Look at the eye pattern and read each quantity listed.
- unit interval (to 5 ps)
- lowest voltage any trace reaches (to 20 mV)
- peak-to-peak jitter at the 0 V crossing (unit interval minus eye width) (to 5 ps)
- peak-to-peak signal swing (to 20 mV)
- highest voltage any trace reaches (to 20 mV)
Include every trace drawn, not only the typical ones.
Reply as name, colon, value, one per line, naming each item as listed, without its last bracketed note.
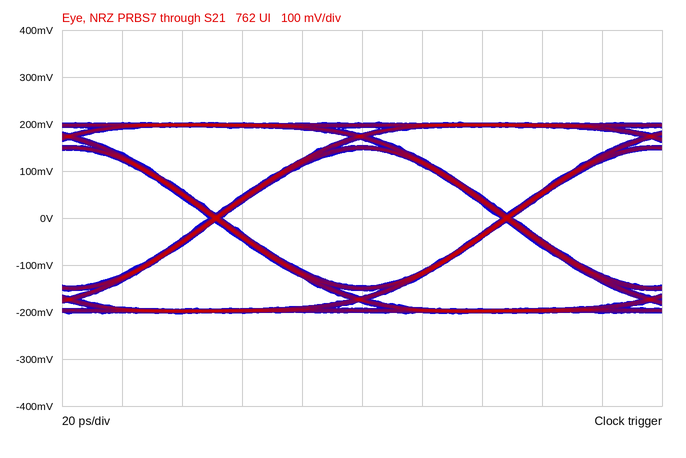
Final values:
unit interval: 95 ps
lowest voltage any trace reaches: -200 mV
peak-to-peak jitter at the 0 V crossing (unit interval minus eye width): 5 ps
peak-to-peak signal swing: 400 mV
highest voltage any trace reaches: 200 mV
